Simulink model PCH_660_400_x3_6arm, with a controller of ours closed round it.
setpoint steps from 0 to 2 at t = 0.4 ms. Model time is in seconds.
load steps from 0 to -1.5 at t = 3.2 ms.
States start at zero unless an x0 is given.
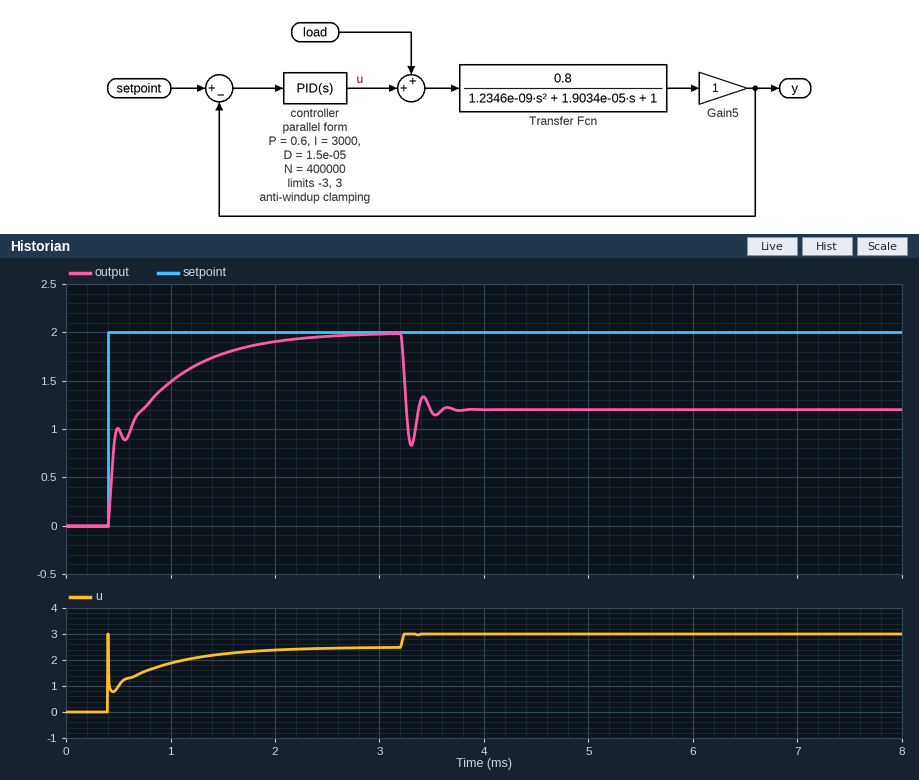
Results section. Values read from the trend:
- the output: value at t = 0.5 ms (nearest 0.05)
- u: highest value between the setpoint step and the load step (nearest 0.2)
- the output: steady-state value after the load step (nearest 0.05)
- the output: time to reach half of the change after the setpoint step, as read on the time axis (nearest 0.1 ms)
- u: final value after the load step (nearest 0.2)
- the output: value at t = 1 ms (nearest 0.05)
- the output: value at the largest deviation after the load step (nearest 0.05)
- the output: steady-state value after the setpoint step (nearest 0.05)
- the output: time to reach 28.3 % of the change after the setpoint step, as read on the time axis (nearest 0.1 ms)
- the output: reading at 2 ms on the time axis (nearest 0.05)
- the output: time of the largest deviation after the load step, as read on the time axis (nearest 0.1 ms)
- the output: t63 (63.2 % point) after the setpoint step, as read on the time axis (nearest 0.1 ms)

1.00
3.0
1.20
0.5 ms
3.0
1.50
0.85
2.00
0.4 ms
1.90
3.3 ms
0.8 ms
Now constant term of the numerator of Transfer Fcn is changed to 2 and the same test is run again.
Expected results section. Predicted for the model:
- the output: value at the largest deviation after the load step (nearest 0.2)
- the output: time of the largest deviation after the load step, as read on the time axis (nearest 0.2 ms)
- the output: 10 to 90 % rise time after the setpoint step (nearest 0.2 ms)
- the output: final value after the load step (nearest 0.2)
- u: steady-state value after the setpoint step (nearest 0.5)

0.4
3.2 ms
0.6 ms
2.0
1.0
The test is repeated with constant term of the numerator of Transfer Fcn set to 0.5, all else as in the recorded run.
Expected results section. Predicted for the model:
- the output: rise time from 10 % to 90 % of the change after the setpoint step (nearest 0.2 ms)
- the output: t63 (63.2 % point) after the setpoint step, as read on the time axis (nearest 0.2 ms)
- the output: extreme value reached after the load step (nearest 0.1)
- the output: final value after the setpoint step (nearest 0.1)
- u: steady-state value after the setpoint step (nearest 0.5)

0.8 ms
0.8 ms
0.4
1.5
3.0
